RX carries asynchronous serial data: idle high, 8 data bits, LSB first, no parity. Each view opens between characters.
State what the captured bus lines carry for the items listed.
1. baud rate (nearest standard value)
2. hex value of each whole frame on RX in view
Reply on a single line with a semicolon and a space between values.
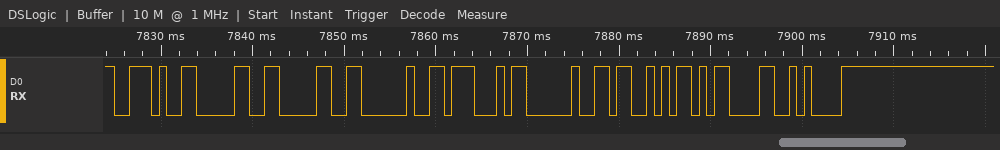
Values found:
1200 baud; 2E, 30, 30, 20, 47, 20, 53, 0D, 0A
